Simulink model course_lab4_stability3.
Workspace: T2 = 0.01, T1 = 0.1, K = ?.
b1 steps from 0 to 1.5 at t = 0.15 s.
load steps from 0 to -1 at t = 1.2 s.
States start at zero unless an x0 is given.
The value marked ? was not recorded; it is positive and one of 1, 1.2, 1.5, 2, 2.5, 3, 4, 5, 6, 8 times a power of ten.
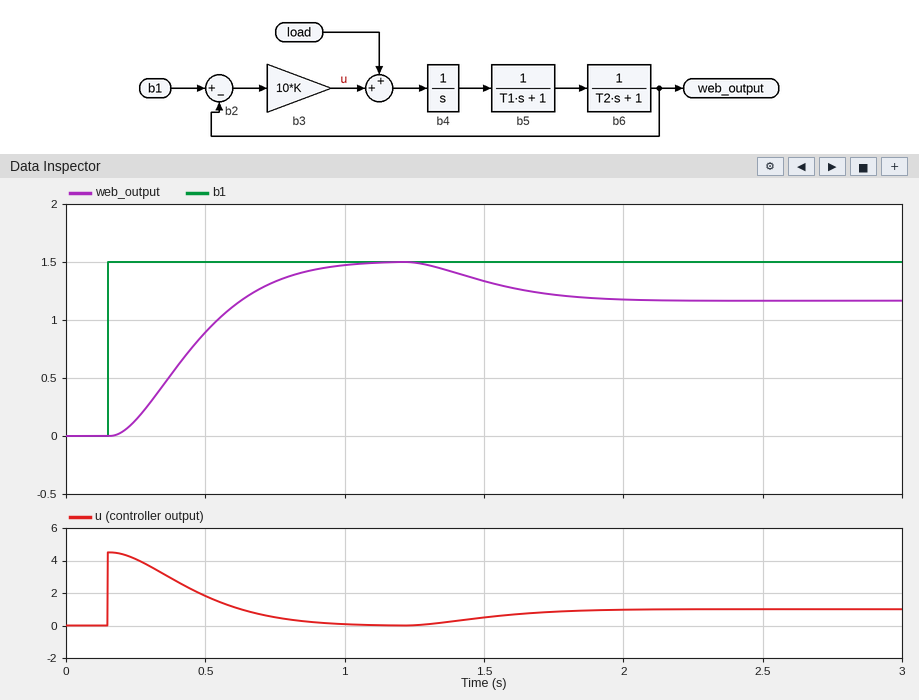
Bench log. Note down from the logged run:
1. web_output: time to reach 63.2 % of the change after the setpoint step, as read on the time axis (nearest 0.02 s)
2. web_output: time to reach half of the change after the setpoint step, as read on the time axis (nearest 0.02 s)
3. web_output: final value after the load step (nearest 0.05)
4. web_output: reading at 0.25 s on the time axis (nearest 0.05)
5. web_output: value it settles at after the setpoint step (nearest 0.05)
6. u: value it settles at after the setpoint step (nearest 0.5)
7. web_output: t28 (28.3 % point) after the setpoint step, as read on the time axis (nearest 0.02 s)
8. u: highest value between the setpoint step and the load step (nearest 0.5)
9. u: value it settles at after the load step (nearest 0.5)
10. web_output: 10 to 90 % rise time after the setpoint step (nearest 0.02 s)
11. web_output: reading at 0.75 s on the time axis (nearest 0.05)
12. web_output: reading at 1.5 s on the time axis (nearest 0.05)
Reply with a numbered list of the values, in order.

1. 0.52 s
2. 0.44 s
3. 1.15
4. 0.15
5. 1.50
6. 0.0
7. 0.34 s
8. 4.5
9. 1.0
10. 0.52 s
11. 1.35
12. 1.35
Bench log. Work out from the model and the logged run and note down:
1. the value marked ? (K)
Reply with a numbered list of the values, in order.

1. 0.3
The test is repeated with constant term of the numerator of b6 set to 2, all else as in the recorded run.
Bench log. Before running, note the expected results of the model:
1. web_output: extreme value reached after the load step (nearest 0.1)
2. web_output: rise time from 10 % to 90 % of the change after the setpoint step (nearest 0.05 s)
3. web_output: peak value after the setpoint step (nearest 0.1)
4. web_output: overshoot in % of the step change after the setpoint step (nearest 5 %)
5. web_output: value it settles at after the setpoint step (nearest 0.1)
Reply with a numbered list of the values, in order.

1. 1.1
2. 0.25 s
3. 1.6
4. 10 %
5. 1.5
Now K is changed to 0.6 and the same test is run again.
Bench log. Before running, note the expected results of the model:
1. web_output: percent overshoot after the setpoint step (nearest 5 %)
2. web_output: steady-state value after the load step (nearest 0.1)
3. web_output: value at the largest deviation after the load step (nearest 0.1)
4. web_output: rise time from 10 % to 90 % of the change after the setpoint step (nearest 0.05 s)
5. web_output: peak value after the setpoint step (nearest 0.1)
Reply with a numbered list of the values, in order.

1. 10 %
2. 1.3
3. 1.3
4. 0.25 s
5. 1.6
